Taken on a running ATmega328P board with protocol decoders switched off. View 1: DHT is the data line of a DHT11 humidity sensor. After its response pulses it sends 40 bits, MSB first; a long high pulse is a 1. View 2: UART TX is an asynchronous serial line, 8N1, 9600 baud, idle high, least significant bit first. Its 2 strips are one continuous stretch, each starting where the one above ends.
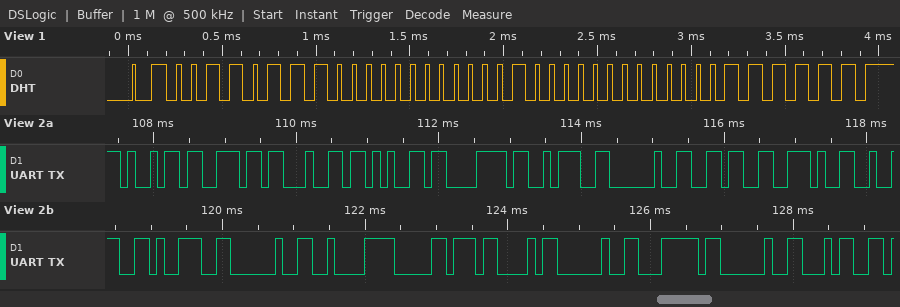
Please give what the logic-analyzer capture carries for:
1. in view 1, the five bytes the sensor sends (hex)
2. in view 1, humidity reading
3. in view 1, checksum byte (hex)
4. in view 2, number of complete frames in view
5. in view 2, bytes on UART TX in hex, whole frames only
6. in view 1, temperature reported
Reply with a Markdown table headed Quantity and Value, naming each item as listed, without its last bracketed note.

| Quantity | Value |
|---|---|
| in view 1, the five bytes the sensor sends | 37 00 08 00 3F |
| in view 1, humidity reading | 55 % |
| in view 1, checksum byte | 0x3F |
| in view 2, number of complete frames in view | 19 |
| in view 2, bytes on UART TX in hex, whole frames only | 69 6E 64 65 78 3A 20 36 2E 32 39 20 C2 B0 43 20 7C 20 34 |
| in view 1, temperature reported | 8.0 °C |
